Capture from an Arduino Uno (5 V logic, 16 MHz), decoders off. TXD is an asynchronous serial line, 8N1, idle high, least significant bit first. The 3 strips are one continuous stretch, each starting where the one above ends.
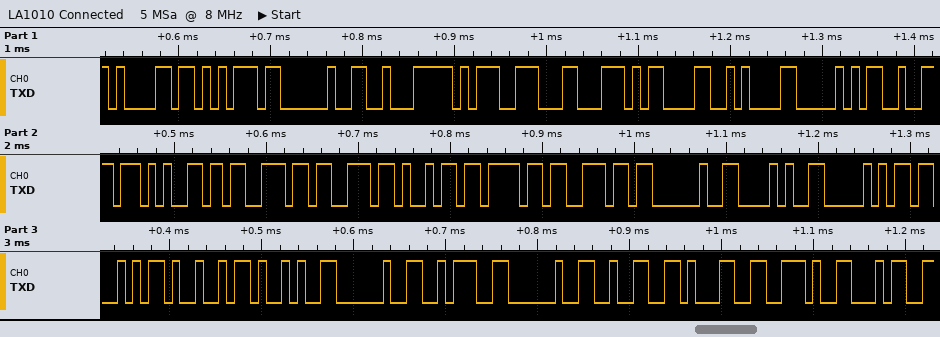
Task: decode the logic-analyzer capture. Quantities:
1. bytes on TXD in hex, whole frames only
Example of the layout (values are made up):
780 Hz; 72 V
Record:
61 75 20 E2 9D 8C 0D 0A 50 72 65 73 73 69 6F 6E 20 28 50 53 49 29 20 3A 20 32 31 2E 34
